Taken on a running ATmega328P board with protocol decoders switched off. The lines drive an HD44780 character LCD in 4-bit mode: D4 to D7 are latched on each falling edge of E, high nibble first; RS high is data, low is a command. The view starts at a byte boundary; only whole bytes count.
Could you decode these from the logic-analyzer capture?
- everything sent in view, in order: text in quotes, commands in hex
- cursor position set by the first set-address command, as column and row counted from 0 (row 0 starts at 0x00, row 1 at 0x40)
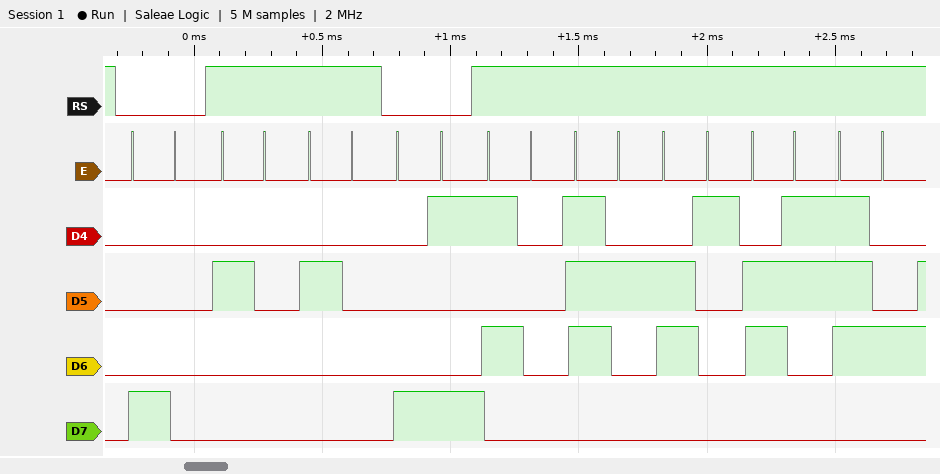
0x80 "  " 0x89 "Pract"
column 0, row 0
